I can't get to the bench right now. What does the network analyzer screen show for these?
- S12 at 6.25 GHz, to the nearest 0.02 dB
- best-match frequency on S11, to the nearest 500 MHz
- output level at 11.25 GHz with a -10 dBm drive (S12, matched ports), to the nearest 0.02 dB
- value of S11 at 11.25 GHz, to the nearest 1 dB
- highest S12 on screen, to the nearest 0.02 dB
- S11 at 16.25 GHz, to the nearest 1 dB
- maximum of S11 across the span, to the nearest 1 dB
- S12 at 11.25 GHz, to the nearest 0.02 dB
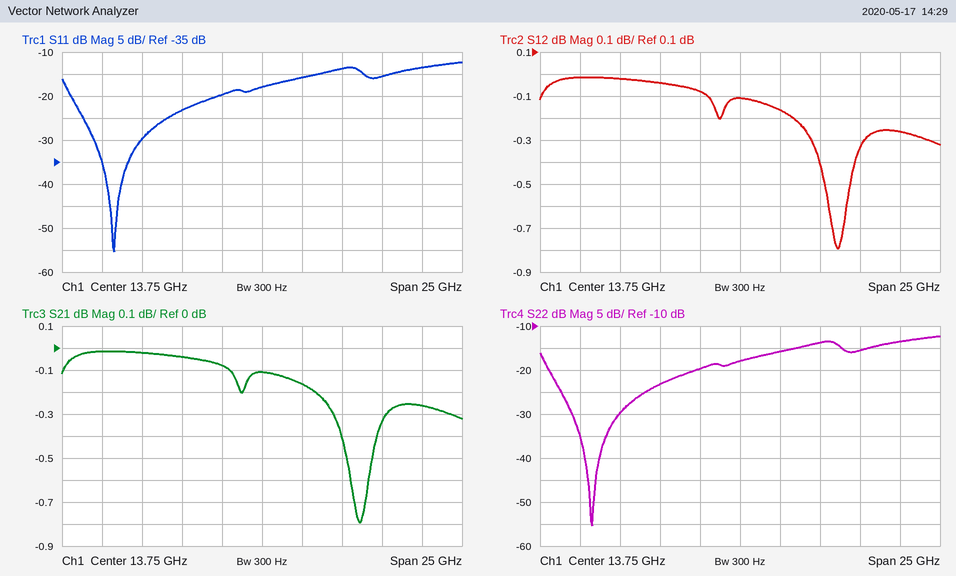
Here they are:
-0.02 dB
4.5 GHz
-10.08 dBm
-20 dB
-0.02 dB
-16 dB
-12 dB
-0.08 dB
